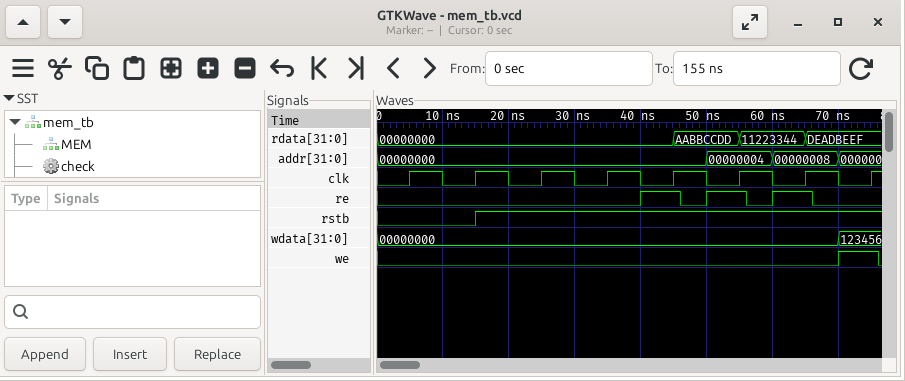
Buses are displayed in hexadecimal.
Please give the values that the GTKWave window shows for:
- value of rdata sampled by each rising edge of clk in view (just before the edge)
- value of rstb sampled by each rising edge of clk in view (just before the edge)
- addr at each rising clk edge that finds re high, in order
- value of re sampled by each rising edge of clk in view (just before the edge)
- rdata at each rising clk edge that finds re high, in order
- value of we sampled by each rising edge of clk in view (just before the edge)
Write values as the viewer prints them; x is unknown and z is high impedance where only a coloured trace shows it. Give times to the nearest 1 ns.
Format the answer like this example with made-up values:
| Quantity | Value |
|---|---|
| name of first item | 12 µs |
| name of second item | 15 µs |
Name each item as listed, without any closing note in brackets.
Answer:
| Quantity | Value |
|---|---|
| value of rdata sampled by each rising edge of clk in view | 00000000, 00000000, 00000000, 00000000, 00000000, AABBCCDD, 11223344, DEADBEEF |
| value of rstb sampled by each rising edge of clk in view | 0 0 1 1 1 1 1 1 |
| addr at each rising clk edge that finds re high, in order | 00000000, 00000004, 00000008 |
| value of re sampled by each rising edge of clk in view | 0 0 0 0 1 1 1 0 |
| rdata at each rising clk edge that finds re high, in order | 00000000, AABBCCDD, 11223344 |
| value of we sampled by each rising edge of clk in view | 0 0 0 0 0 0 0 1 |
